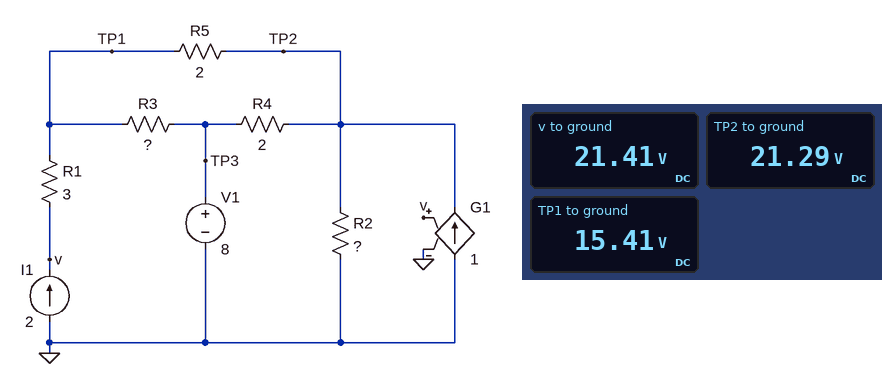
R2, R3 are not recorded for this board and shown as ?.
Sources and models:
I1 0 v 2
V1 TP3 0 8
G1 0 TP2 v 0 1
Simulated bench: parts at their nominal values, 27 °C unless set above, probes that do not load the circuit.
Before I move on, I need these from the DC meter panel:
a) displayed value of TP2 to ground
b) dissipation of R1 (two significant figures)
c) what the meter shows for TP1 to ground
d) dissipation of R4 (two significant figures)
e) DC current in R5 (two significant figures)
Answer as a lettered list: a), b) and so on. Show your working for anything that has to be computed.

a) 21.29 V
b) (21.41 V - 15.41 V)^2 / 3 Ω = 12 W
c) 15.41 V
d) (21.29 V - 8 V)^2 / 2 Ω = 88 W
e) (21.29 V - 15.41 V) / 2 Ω = 2.9 A
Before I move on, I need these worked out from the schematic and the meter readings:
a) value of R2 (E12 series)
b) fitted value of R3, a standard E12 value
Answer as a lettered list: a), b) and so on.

a) 1.8 Ω
b) 1.5 Ω
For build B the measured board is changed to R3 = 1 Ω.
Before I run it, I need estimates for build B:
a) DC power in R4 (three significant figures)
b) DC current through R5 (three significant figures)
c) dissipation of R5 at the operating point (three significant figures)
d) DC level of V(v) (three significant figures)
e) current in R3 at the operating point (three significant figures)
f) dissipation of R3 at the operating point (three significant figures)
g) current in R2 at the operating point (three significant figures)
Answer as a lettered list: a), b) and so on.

a) 59.9 W
b) 2.98 A
c) 17.8 W
d) 19.0 V
e) 4.98 A
f) 24.8 W
g) 10.5 A
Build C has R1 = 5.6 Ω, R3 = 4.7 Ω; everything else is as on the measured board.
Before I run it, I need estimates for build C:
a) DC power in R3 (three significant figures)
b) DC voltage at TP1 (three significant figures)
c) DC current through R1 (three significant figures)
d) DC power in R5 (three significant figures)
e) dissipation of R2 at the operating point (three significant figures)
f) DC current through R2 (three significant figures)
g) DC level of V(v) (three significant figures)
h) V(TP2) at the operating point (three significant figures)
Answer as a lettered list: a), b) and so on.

a) 182 W
b) 37.2 V
c) 2.00 A
d) 35.6 W
e) 1.16 kW
f) 25.4 A
g) 48.4 V
h) 45.7 V
